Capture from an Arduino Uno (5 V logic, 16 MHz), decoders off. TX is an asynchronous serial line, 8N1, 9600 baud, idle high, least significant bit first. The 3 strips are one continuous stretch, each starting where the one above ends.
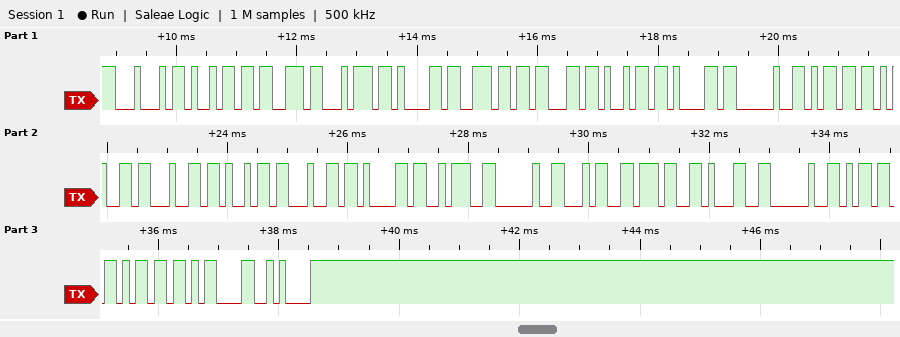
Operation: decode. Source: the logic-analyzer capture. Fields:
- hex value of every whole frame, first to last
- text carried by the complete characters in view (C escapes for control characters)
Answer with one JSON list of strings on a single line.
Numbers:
["0x44 0x69 0x73 0x74 0x61 0x6E 0x63 0x69 0x61 0x20 0x6D 0x65 0x64 0x69 0x64 0x61 0x3A 0x20 0x34 0x37 0x31 0x20 0x6D 0x6D 0x0D 0x0A", "\"Distancia medida: 471 mm\\r\\n\""]
